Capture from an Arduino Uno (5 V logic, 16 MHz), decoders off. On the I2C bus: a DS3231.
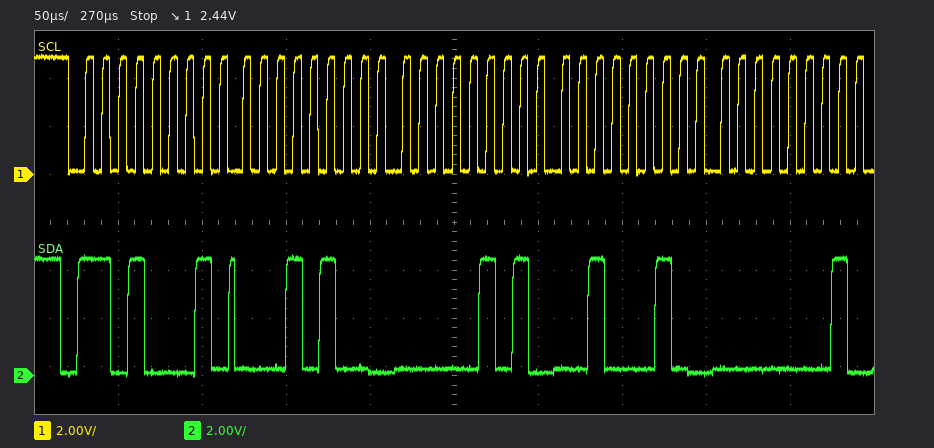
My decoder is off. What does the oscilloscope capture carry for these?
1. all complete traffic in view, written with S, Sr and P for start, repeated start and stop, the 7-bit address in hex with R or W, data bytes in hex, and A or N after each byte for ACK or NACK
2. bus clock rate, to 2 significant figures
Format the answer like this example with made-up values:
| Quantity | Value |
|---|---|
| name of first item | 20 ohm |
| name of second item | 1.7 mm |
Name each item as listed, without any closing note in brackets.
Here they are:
| Quantity | Value |
|---|---|
| all complete traffic in view, written with S, Sr and P for start, repeated start and stop, the 7-bit address in hex with R or W, data bytes in hex, and A or N after each byte for ACK or NACK | S 68R A 14 A 05 A 22 A 01 A |
| bus clock rate, to 2 significant figures | 100 kHz |
